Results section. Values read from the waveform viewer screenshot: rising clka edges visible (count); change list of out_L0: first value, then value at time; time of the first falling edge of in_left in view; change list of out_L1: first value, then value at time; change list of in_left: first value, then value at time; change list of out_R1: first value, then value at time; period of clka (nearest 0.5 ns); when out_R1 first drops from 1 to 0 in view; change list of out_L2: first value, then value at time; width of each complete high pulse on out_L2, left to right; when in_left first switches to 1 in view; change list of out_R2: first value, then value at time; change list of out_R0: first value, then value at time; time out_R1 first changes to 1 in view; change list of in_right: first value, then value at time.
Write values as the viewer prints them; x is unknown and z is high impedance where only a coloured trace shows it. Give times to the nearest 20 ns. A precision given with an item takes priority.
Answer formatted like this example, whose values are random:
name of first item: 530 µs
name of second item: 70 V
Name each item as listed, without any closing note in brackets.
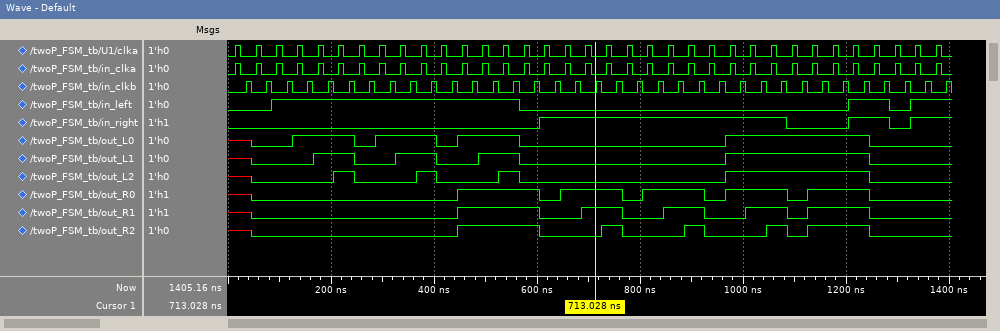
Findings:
rising clka edges visible: 35
change list of out_L0: first value, then value at time: x, 0 at 40 ns, 1 at 120 ns, 0 at 240 ns, 1 at 280 ns, 0 at 400 ns, 1 at 440 ns, 0 at 560 ns, 1 at 960 ns, 0 at 1240 ns
time of the first falling edge of in_left in view: 560 ns
change list of out_L1: first value, then value at time: x, 0 at 40 ns, 1 at 160 ns, 0 at 240 ns, 1 at 320 ns, 0 at 400 ns, 1 at 480 ns, 0 at 560 ns, 1 at 960 ns, 0 at 1240 ns
change list of in_left: first value, then value at time: 0, 1 at 80 ns, 0 at 560 ns, 1 at 1200 ns, 0 at 1280 ns, 1 at 1320 ns
change list of out_R1: first value, then value at time: x, 0 at 40 ns, 1 at 440 ns, 0 at 600 ns, 1 at 680 ns, 0 at 760 ns, 1 at 840 ns, 0 at 920 ns, 1 at 1000 ns, 0 at 1080 ns, 1 at 1120 ns, 0 at 1240 ns
period of clka: 40 ns
when out_R1 first drops from 1 to 0 in view: 600 ns
change list of out_L2: first value, then value at time: x, 0 at 40 ns, 1 at 200 ns, 0 at 240 ns, 1 at 360 ns, 0 at 400 ns, 1 at 520 ns, 0 at 560 ns, 1 at 960 ns, 0 at 1240 ns
width of each complete high pulse on out_L2, left to right: 40 ns, 40 ns, 40 ns, 280 ns
when in_left first switches to 1 in view: 80 ns
change list of out_R2: first value, then value at time: x, 0 at 40 ns, 1 at 440 ns, 0 at 600 ns, 1 at 720 ns, 0 at 760 ns, 1 at 880 ns, 0 at 920 ns, 1 at 1040 ns, 0 at 1080 ns, 1 at 1120 ns, 0 at 1240 ns
change list of out_R0: first value, then value at time: x, 0 at 40 ns, 1 at 440 ns, 0 at 600 ns, 1 at 640 ns, 0 at 760 ns, 1 at 800 ns, 0 at 920 ns, 1 at 960 ns, 0 at 1080 ns, 1 at 1120 ns, 0 at 1240 ns
time out_R1 first changes to 1 in view: 440 ns
change list of in_right: first value, then value at time: 0, 1 at 600 ns, 0 at 1080 ns, 1 at 1200 ns, 0 at 1280 ns, 1 at 1320 ns
